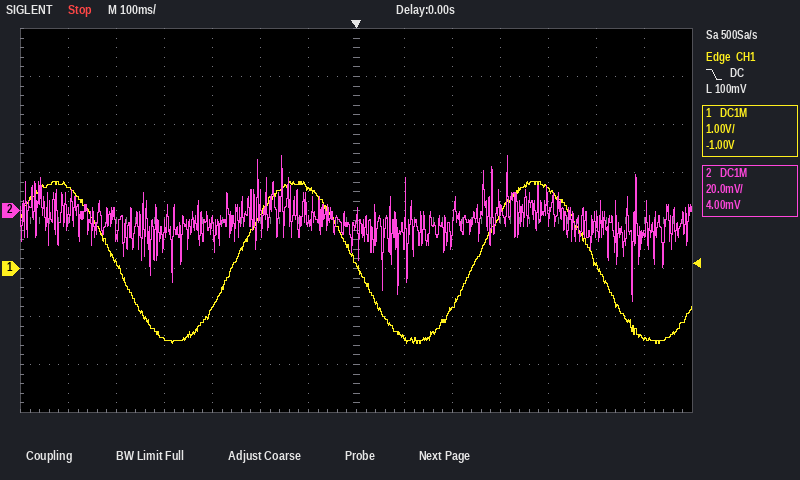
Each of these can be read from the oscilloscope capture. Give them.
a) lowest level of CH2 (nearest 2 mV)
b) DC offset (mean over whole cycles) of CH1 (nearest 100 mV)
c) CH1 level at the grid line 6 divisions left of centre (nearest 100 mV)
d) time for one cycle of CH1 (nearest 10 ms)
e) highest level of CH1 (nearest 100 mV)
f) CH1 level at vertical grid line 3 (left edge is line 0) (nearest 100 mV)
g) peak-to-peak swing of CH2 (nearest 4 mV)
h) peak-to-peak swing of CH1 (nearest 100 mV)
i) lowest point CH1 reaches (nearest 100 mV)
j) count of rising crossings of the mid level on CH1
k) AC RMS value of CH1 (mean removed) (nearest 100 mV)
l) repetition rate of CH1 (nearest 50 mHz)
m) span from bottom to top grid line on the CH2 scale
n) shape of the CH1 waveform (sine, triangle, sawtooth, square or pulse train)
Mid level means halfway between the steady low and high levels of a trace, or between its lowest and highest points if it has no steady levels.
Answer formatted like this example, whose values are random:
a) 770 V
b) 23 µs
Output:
a) -38 mV
b) 100 mV
c) 1.7 V
d) 500 ms
e) 1.8 V
f) -1.5 V
g) 60 mV
h) 3.4 V
i) -1.6 V
j) 2
k) 1.2 V
l) 2.00 Hz
m) 160 mV
n) sine
